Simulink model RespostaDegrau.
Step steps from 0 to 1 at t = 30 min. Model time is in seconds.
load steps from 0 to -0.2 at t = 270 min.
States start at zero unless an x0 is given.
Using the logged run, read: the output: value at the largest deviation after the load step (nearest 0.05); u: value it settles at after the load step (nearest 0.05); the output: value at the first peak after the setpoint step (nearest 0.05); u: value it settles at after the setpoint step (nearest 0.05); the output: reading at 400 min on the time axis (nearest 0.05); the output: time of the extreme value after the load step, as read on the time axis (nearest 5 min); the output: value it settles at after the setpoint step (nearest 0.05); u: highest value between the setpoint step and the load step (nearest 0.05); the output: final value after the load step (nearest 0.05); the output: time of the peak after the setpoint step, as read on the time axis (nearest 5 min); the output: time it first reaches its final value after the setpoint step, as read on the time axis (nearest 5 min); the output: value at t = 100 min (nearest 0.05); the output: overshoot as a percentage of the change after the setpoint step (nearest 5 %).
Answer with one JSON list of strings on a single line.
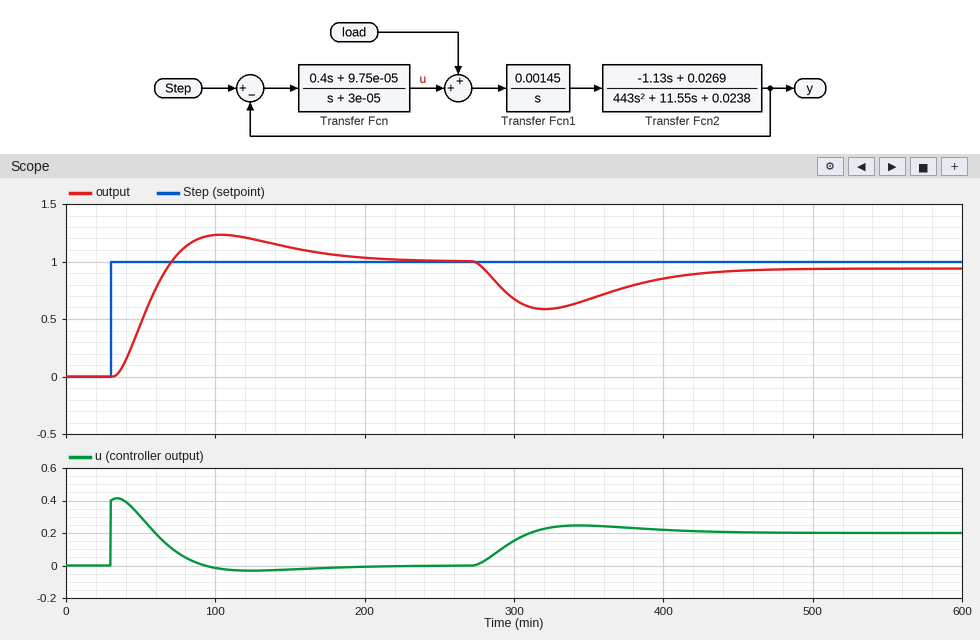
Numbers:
["0.60", "0.20", "1.25", "0.00", "0.85", "320 min", "1.00", "0.40", "0.95", "105 min", "70 min", "1.25", "25 %"]
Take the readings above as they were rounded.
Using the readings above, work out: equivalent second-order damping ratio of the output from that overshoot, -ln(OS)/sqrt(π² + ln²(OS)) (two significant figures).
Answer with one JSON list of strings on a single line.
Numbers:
["0.40"]
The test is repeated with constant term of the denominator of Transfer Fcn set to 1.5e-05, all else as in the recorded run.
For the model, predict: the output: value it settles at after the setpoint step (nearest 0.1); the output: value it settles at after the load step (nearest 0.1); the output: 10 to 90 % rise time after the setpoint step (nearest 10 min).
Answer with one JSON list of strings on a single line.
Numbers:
["1.0", "1.0", "30 min"]
